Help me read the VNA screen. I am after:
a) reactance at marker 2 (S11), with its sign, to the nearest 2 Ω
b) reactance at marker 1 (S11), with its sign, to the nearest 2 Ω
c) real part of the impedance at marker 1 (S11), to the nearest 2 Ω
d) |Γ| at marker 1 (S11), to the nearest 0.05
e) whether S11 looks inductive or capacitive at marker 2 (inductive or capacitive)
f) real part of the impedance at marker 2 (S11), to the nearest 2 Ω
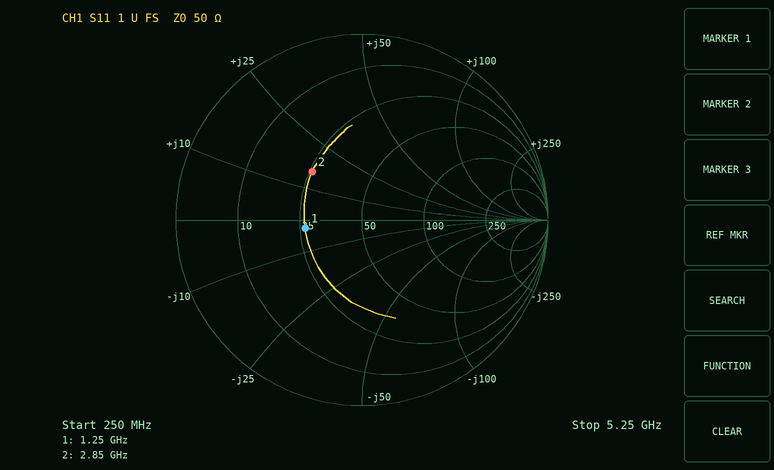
+16 Ω
-2 Ω
26 Ω
0.30
inductive
26 Ω
